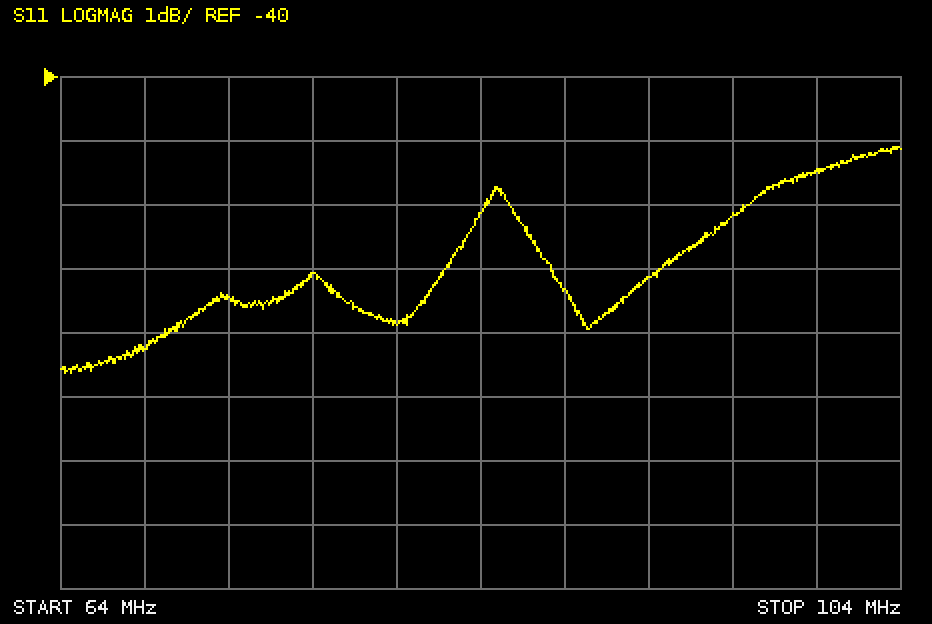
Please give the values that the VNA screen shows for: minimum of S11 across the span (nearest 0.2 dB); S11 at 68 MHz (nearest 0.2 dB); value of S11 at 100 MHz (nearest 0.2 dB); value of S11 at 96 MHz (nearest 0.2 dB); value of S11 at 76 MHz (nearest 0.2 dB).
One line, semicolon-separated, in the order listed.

-44.6 dB; -44.2 dB; -41.4 dB; -42.2 dB; -43.0 dB
